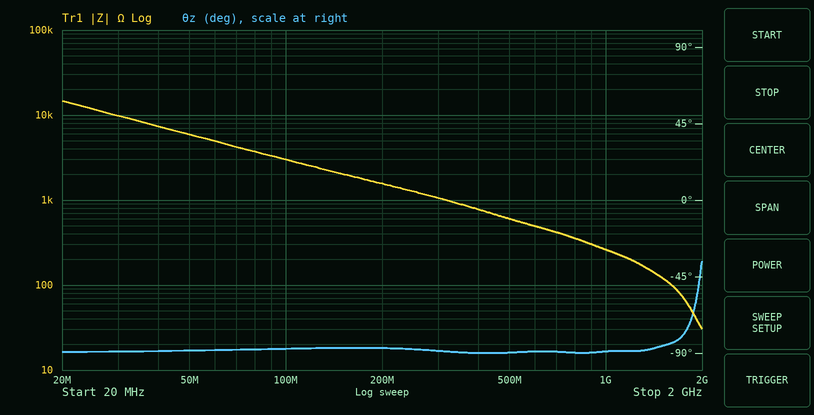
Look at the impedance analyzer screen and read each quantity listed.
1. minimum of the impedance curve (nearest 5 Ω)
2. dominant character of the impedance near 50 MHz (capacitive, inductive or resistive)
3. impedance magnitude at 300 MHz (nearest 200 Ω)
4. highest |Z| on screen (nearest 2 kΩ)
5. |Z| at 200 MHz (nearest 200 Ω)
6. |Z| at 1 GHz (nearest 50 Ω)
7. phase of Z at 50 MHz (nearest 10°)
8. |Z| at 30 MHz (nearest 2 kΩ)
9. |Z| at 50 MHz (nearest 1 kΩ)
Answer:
30 Ω
capacitive
1.0 kΩ
14 kΩ
1.6 kΩ
250 Ω
-90°
10 kΩ
6 kΩ
